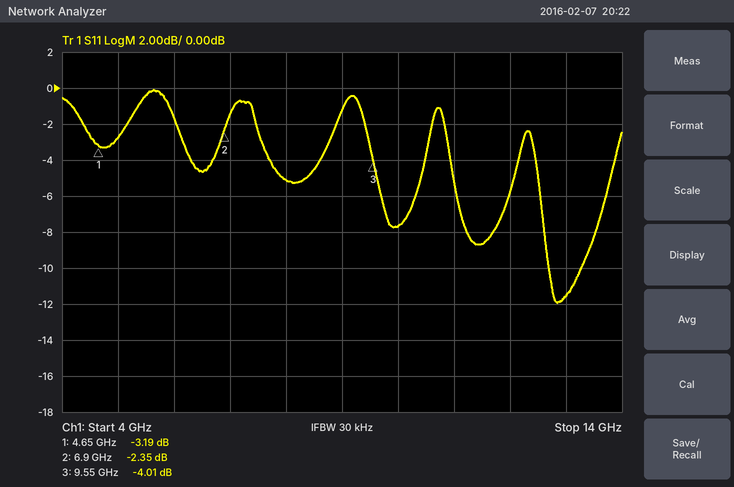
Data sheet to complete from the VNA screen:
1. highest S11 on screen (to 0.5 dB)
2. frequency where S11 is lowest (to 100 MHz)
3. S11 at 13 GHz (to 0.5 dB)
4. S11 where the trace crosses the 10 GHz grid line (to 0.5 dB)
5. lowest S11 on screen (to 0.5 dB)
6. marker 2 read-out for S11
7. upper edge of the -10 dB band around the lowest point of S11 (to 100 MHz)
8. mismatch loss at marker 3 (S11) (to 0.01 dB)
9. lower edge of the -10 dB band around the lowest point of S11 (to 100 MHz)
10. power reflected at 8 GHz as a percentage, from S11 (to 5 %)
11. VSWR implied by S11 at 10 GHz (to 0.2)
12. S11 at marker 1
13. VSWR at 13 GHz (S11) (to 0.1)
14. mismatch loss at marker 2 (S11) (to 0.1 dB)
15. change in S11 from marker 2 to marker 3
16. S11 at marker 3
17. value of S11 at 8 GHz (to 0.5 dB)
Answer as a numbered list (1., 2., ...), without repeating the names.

1. 0.0 dB
2. 12.8 GHz
3. -11.5 dB
4. -7.5 dB
5. -12.0 dB
6. -2.35 dB
7. 13.3 GHz
8. 2.20 dB
9. 12.7 GHz
10. 30 %
11. 2.4
12. -3.19 dB
13. 1.7
14. 3.8 dB
15. -1.66 dB
16. -4.01 dB
17. -5.0 dB
